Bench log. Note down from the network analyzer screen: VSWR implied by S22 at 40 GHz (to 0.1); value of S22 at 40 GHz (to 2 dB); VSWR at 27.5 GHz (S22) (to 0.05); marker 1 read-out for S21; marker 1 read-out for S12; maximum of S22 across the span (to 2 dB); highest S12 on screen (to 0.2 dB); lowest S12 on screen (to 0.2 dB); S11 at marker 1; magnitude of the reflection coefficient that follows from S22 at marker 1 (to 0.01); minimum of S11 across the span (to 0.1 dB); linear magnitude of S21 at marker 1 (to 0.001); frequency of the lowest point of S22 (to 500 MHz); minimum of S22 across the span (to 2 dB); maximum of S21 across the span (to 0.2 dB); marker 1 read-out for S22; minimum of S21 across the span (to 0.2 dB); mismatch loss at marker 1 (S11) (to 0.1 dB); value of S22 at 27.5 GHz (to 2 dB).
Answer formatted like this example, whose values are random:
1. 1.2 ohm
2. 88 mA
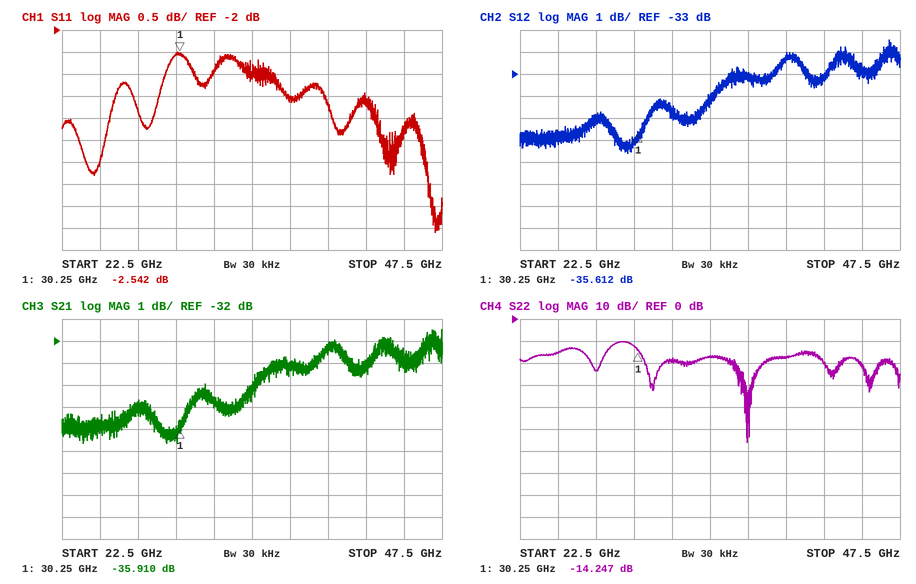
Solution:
1. 1.3
2. -18 dB
3. 1.15
4. -35.910 dB
5. -35.612 dB
6. -10 dB
7. -31.4 dB
8. -36.6 dB
9. -2.542 dB
10. 0.19
11. -6.6 dB
12. 0.016
13. 37.5 GHz
14. -56 dB
15. -31.4 dB
16. -14.247 dB
17. -36.6 dB
18. 3.5 dB
19. -24 dB
